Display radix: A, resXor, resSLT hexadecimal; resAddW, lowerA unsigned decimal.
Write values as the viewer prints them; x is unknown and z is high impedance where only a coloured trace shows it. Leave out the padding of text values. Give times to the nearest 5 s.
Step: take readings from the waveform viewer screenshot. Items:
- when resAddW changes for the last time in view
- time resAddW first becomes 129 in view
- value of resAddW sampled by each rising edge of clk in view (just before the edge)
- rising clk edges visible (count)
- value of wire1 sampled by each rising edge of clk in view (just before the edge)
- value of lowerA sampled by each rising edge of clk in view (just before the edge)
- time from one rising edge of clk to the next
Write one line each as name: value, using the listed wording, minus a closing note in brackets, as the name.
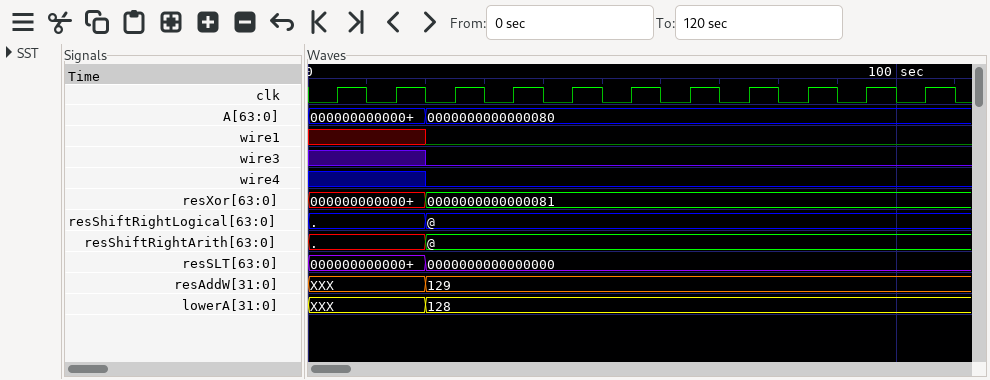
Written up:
when resAddW changes for the last time in view: 20 s
time resAddW first becomes 129 in view: 20 s
value of resAddW sampled by each rising edge of clk in view: XXX, XXX, 129, 129, 129, 129, 129, 129, 129, 129, 129
rising clk edges visible: 11
value of wire1 sampled by each rising edge of clk in view: x x 0 0 0 0 0 0 0 0 0
value of lowerA sampled by each rising edge of clk in view: XXX, XXX, 128, 128, 128, 128, 128, 128, 128, 128, 128
time from one rising edge of clk to the next: 10 s
